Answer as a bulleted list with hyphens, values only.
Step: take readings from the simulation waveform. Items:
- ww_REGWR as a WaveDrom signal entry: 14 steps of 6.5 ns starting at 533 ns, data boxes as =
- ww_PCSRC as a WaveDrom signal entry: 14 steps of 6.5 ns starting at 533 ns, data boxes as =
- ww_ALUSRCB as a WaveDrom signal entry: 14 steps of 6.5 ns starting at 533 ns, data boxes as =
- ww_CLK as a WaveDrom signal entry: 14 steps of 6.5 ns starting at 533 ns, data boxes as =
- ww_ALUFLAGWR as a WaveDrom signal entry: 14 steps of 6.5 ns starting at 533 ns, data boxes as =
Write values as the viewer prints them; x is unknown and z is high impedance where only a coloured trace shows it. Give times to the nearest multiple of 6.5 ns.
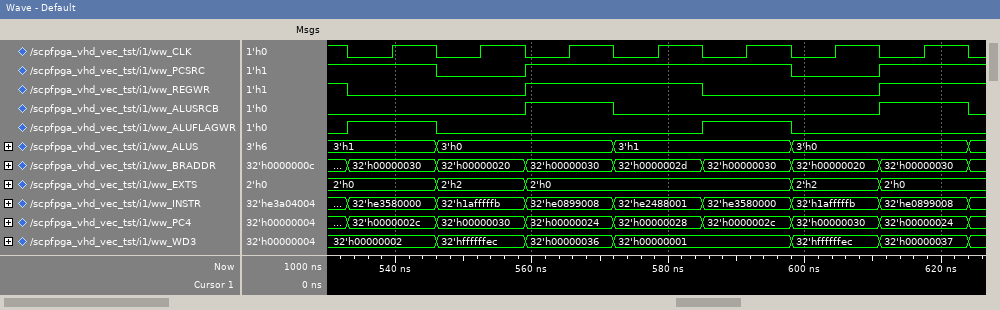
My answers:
- {name: 'ww_REGWR', wave: '0...1...0...1.'}
- {name: 'ww_PCSRC', wave: '1.0.1.....0.1.'}
- {name: 'ww_ALUSRCB', wave: '0...1.0.....1.'}
- {name: 'ww_CLK', wave: '01010101010101'}
- {name: 'ww_ALUFLAGWR', wave: '1.0.....1.0...'}
